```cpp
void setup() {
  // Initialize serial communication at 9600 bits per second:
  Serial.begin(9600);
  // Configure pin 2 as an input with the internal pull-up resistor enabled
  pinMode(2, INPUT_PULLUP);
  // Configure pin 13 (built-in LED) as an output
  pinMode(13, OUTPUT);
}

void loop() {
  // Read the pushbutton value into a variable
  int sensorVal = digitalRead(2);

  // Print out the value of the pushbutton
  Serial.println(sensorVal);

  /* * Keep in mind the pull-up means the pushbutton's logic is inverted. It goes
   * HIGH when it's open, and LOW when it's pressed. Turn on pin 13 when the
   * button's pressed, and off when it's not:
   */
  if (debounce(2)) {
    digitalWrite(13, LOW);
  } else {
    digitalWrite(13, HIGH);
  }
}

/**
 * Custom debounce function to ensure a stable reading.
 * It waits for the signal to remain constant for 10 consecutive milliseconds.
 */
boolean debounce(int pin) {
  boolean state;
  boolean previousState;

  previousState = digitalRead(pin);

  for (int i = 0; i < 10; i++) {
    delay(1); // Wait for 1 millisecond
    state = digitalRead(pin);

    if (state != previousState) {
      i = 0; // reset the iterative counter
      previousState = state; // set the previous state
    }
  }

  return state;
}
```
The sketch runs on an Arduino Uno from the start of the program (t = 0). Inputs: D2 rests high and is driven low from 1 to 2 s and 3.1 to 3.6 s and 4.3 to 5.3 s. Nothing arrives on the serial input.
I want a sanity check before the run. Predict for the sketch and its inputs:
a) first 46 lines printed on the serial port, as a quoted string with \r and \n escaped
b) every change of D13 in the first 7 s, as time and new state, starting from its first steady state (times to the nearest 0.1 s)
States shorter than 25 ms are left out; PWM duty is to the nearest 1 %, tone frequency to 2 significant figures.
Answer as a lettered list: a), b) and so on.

a) "1\r\n1\r\n1\r\n1\r\n1\r\n1\r\n1\r\n1\r\n1\r\n1\r\n1\r\n1\r\n1\r\n1\r\n1\r\n1\r\n1\r\n1\r\n1\r\n1\r\n1\r\n1\r\n1\r\n1\r\n1\r\n1\r\n1\r\n1\r\n1\r\n1\r\n1\r\n1\r\n1\r\n1\r\n1\r\n1\r\n1\r\n1\r\n1\r\n1\r\n1\r\n1\r\n1\r\n1\r\n1\r\n1\r\n"
b) 0 s low; 1 s high; 2 s low; 3.1 s high; 3.6 s low; 4.3 s high; 5.3 s low
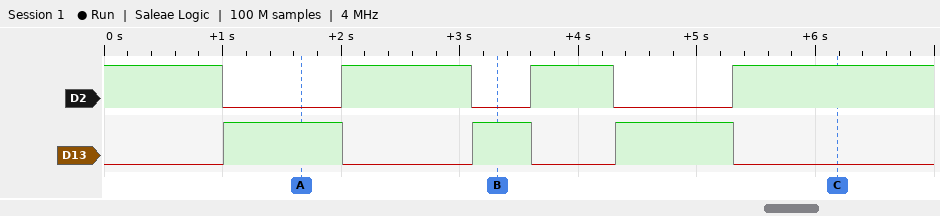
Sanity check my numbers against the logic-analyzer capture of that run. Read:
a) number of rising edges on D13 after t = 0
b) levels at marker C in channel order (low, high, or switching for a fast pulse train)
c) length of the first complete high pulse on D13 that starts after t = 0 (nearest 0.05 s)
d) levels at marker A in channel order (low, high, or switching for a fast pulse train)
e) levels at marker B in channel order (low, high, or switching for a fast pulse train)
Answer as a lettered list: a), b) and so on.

a) 3
b) D2 high, D13 low
c) 1.00 s
d) D2 low, D13 high
e) D2 low, D13 high
